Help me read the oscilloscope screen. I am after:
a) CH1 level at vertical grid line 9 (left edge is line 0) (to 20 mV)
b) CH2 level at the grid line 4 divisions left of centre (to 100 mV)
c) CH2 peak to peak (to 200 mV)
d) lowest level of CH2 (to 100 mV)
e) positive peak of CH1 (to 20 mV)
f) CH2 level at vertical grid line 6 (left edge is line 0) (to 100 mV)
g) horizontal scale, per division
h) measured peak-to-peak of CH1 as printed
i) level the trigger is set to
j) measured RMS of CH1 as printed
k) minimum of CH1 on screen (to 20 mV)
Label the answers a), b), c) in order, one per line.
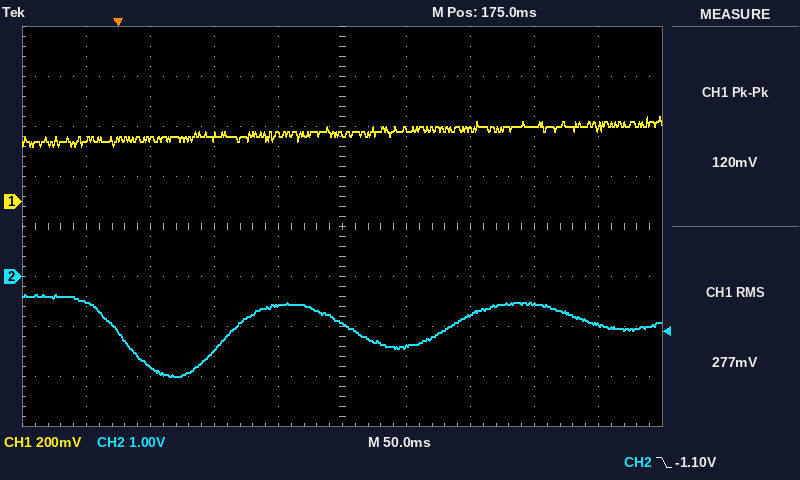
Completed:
a) 300 mV
b) -500 mV
c) 1.6 V
d) -2.0 V
e) 340 mV
f) -1.4 V
g) 50 ms
h) 120 mV
i) -1.10 V
j) 277 mV
k) 220 mV
